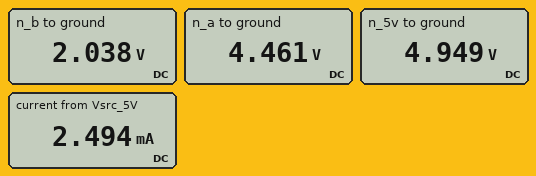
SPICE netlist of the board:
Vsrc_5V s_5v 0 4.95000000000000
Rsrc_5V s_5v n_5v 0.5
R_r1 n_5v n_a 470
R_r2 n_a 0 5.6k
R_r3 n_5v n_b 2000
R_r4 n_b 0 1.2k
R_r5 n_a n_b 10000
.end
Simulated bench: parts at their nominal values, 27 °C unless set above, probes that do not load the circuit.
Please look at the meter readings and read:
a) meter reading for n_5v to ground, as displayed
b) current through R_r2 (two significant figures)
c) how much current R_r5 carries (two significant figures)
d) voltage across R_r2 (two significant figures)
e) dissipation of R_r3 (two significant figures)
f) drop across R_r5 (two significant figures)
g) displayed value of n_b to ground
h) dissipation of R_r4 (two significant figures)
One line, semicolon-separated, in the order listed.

4.949 V; 800 µA; 240 µA; 4.5 V; 4.2 mW; 2.4 V; 2.038 V; 3.5 mW
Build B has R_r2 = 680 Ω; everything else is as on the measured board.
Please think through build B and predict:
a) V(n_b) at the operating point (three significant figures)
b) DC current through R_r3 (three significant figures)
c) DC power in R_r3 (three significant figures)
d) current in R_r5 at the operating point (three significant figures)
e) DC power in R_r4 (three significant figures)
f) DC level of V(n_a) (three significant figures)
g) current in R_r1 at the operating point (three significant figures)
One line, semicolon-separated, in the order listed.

1.93 V; 1.51 mA; 4.56 mW; 97.0 µA; 3.10 mW; 2.90 V; 4.36 mA
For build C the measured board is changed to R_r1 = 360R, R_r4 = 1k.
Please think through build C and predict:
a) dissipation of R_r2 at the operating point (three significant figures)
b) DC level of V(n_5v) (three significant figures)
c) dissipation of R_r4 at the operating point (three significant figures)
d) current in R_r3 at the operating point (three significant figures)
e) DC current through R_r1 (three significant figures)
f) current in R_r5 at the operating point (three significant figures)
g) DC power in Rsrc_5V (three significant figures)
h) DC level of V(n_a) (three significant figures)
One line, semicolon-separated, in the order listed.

3.71 mW; 4.95 V; 3.35 mW; 1.56 mA; 1.09 mA; 273 µA; 3.50 µW; 4.56 V
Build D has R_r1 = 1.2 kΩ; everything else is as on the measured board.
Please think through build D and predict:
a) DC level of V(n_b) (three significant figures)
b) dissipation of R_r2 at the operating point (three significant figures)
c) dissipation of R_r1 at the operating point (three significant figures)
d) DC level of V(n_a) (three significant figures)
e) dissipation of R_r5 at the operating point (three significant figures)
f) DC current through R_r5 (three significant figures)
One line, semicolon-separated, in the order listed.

2.00 V; 2.70 mW; 937 µW; 3.89 V; 358 µW; 189 µA
